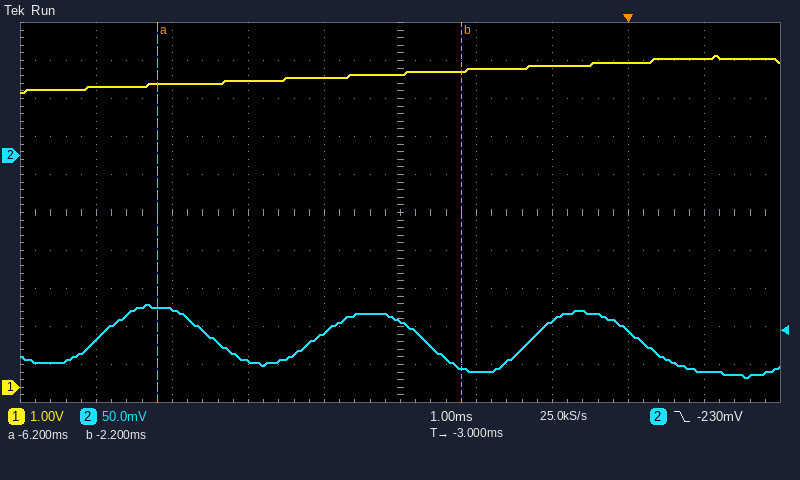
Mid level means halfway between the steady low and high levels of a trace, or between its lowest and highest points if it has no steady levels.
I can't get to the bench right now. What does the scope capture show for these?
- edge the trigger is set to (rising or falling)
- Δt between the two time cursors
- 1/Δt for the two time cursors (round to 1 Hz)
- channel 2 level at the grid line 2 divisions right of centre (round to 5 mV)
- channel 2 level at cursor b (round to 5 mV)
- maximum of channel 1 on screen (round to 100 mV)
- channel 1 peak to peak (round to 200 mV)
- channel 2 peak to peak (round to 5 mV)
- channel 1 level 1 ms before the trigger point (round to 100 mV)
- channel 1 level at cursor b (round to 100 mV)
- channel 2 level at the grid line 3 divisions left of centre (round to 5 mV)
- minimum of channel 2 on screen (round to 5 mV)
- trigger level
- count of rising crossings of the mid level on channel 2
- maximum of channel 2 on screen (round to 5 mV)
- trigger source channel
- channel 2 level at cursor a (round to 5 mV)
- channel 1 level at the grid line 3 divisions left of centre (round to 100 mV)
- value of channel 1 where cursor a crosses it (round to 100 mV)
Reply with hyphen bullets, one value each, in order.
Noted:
- falling
- 4.0 ms
- 250 Hz
- -215 mV
- -280 mV
- 8.7 V
- 1.0 V
- 95 mV
- 8.5 V
- 8.3 V
- -200 mV
- -290 mV
- -230 mV
- 3
- -195 mV
- channel 2
- -200 mV
- 8.0 V
- 8.0 V
